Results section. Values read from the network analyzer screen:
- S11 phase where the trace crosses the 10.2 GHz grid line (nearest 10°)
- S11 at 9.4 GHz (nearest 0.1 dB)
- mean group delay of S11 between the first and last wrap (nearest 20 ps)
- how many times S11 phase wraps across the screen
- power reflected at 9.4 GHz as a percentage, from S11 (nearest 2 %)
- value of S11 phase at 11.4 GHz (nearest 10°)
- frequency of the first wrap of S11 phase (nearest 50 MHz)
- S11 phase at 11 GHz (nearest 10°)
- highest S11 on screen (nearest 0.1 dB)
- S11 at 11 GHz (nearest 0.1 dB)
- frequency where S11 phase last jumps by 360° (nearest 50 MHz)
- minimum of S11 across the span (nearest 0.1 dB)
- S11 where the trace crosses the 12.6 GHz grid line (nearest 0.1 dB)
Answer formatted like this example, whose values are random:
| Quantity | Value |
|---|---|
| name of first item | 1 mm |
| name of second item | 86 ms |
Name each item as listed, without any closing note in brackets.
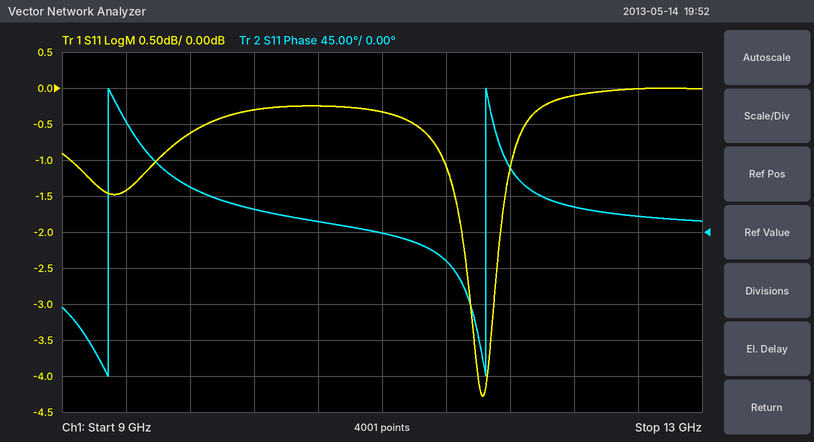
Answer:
| Quantity | Value |
|---|---|
| S11 phase where the trace crosses the 10.2 GHz grid line | 30° |
| S11 at 9.4 GHz | -1.4 dB |
| mean group delay of S11 between the first and last wrap | 420 ps |
| how many times S11 phase wraps across the screen | 2 |
| power reflected at 9.4 GHz as a percentage, from S11 | 72 % |
| value of S11 phase at 11.4 GHz | -40° |
| frequency of the first wrap of S11 phase | 9.30 GHz |
| S11 phase at 11 GHz | 0° |
| highest S11 on screen | 0.0 dB |
| S11 at 11 GHz | -0.3 dB |
| frequency where S11 phase last jumps by 360° | 11.65 GHz |
| minimum of S11 across the span | -4.3 dB |
| S11 where the trace crosses the 12.6 GHz grid line | 0.0 dB |
